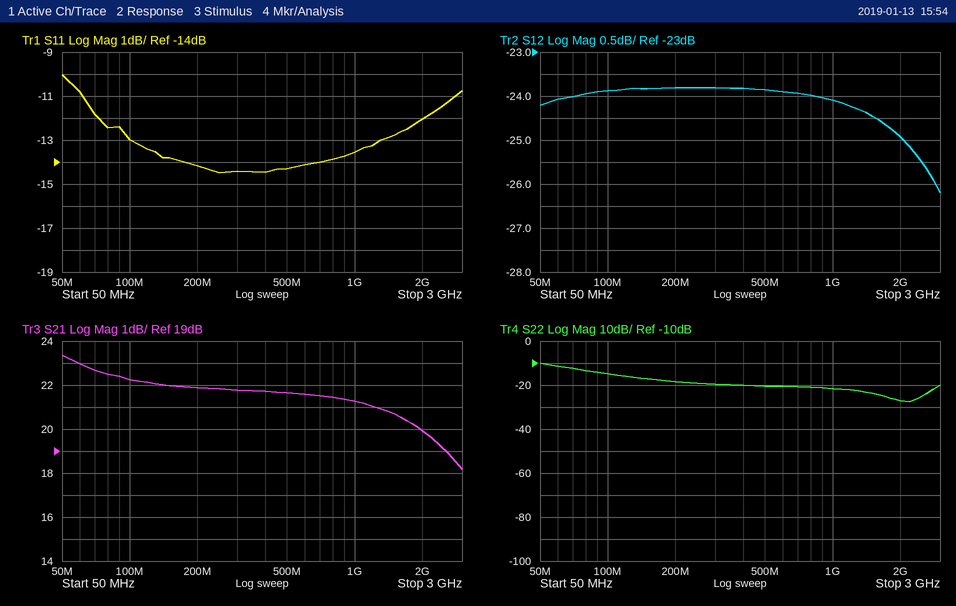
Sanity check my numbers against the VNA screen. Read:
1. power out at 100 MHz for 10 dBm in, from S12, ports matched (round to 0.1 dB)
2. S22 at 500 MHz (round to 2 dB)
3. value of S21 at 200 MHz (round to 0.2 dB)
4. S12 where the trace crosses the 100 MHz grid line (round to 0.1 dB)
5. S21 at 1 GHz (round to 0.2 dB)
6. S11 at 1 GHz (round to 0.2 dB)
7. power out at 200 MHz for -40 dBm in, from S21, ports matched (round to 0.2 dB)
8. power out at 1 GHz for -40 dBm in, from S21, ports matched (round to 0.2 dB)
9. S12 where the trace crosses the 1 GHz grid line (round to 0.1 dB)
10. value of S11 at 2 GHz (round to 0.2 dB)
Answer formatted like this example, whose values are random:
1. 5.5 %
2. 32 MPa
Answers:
1. -13.9 dBm
2. -20 dB
3. 21.8 dB
4. -23.9 dB
5. 21.2 dB
6. -13.6 dB
7. -18.2 dBm
8. -18.8 dBm
9. -24.1 dB
10. -12.0 dB
